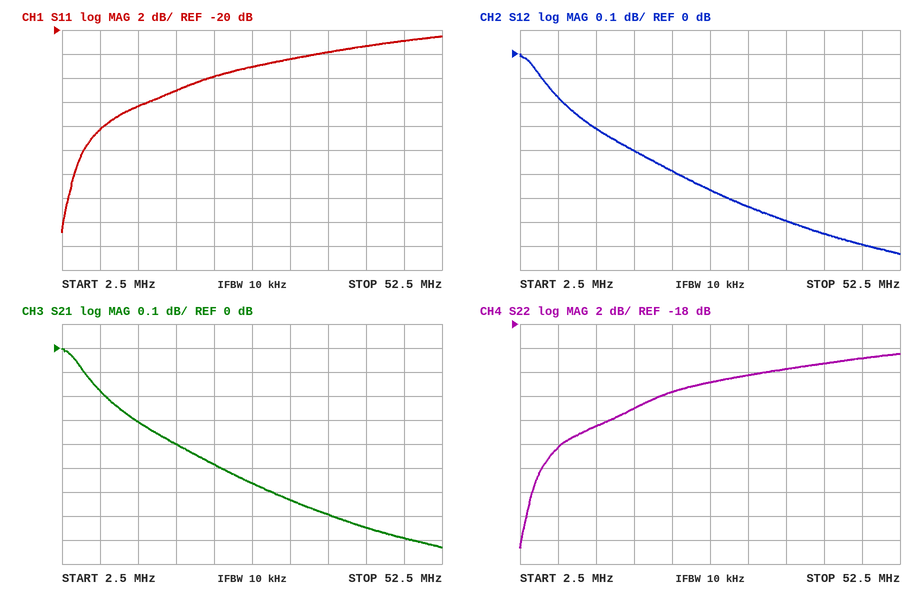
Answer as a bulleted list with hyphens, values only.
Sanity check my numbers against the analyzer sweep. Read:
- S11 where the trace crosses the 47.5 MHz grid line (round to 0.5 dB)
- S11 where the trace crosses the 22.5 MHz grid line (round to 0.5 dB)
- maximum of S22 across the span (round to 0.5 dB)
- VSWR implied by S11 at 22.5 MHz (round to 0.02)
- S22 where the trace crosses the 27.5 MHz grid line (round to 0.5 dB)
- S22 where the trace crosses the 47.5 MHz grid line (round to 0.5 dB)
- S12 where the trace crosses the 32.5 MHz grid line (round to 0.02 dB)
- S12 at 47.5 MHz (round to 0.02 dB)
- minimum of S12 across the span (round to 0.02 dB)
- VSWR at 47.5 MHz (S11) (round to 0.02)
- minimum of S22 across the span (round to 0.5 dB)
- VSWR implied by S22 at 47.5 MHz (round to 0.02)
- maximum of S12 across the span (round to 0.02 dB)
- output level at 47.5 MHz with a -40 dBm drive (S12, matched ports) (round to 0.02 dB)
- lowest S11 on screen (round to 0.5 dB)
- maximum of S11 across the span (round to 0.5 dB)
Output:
- -21.0 dB
- -24.0 dB
- -20.5 dB
- 1.14
- -23.0 dB
- -21.0 dB
- -0.64 dB
- -0.80 dB
- -0.84 dB
- 1.20
- -36.5 dB
- 1.20
- 0.00 dB
- -40.80 dBm
- -37.0 dB
- -20.5 dB
